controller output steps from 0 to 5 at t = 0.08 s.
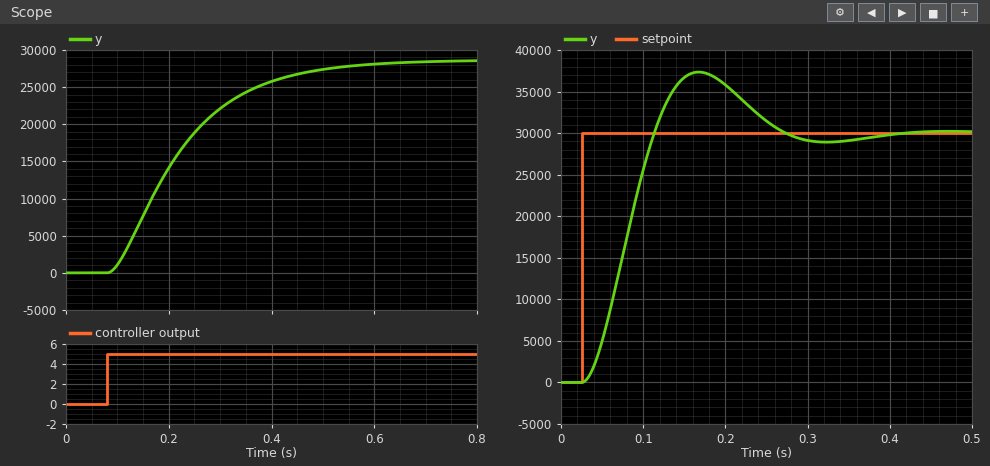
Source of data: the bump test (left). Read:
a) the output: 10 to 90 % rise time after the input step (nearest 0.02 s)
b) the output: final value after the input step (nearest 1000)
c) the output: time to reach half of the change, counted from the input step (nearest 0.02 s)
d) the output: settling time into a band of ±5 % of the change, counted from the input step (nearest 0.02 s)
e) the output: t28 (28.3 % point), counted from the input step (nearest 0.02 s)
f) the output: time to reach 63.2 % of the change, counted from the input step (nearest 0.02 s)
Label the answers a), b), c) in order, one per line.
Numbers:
a) 0.28 s
b) 29000
c) 0.12 s
d) 0.40 s
e) 0.08 s
f) 0.16 s
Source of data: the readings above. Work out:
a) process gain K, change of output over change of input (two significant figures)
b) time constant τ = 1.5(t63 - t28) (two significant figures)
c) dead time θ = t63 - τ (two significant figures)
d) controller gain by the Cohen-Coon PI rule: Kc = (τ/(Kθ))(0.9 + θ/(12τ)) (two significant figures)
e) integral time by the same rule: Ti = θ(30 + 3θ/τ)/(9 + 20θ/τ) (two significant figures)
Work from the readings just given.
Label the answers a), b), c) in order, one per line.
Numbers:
a) 5800
b) 0.12 s
c) 0.040 s
d) 0.00048
e) 0.079 s
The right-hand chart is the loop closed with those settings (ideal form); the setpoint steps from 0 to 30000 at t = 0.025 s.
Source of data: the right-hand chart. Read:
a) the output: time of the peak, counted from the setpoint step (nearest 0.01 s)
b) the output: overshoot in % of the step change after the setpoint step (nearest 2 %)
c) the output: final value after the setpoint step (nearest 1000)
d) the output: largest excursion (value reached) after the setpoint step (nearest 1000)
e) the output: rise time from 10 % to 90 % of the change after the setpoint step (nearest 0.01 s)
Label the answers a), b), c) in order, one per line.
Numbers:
a) 0.14 s
b) 24 %
c) 30000
d) 37000
e) 0.06 s
